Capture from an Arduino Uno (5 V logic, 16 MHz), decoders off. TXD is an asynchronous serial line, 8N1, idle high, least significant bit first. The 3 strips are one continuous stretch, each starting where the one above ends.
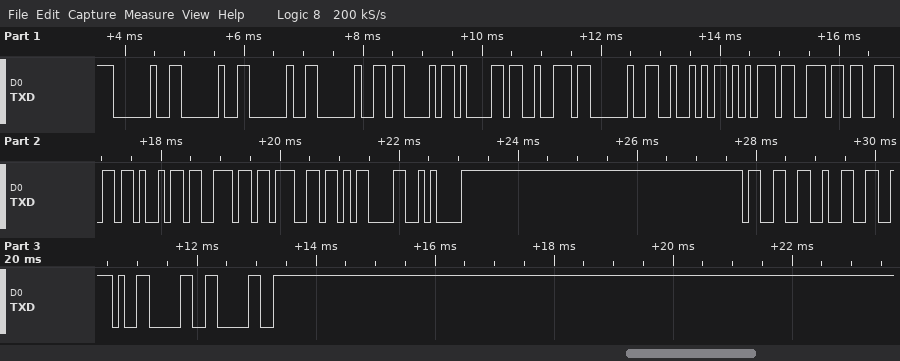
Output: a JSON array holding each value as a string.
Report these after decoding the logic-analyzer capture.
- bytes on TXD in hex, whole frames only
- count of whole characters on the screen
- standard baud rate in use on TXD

["20 20 20 20 43 61 72 20 52 75 6E 6E 69 6E 67 0D 0A 33 32 2E 30 30", "22", "9600 baud"]
